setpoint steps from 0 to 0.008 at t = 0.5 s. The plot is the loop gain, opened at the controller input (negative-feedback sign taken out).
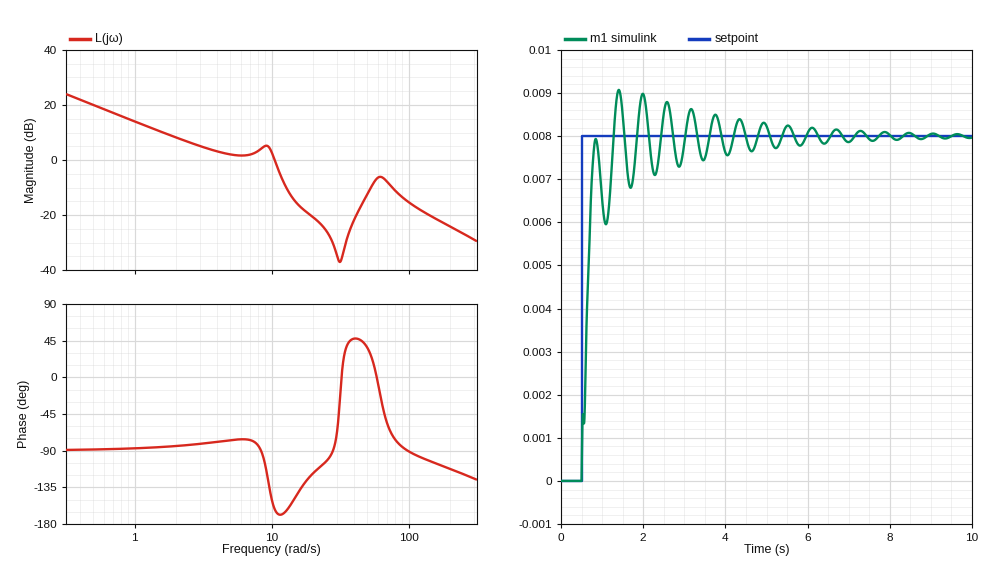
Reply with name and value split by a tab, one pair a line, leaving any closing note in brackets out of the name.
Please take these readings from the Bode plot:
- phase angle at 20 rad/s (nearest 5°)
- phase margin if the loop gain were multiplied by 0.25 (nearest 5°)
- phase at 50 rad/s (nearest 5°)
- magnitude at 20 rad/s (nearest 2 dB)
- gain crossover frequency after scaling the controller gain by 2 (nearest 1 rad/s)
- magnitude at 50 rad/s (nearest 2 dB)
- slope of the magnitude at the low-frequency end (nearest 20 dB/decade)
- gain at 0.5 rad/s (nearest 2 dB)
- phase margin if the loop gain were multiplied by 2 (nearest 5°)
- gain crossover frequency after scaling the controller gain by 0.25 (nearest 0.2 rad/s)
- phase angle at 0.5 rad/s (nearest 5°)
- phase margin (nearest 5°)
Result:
phase angle at 20 rad/s	-120°
phase margin if the loop gain were multiplied by 0.25	95°
phase at 50 rad/s	35°
magnitude at 20 rad/s	-20 dB
gain crossover frequency after scaling the controller gain by 2	12 rad/s
magnitude at 50 rad/s	-12 dB
slope of the magnitude at the low-frequency end	-20 dB/decade
gain at 0.5 rad/s	20 dB
phase margin if the loop gain were multiplied by 2	10°
gain crossover frequency after scaling the controller gain by 0.25	1.2 rad/s
phase angle at 0.5 rad/s	-90°
phase margin	20°
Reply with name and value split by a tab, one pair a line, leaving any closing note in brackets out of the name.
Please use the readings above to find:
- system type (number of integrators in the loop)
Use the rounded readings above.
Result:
system type	1
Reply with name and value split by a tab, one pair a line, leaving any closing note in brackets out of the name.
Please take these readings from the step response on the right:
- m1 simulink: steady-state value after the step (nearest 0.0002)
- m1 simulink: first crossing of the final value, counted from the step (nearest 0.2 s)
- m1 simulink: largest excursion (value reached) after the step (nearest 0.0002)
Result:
m1 simulink: steady-state value after the step	0.0080
m1 simulink: first crossing of the final value, counted from the step	0.8 s
m1 simulink: largest excursion (value reached) after the step	0.0090
